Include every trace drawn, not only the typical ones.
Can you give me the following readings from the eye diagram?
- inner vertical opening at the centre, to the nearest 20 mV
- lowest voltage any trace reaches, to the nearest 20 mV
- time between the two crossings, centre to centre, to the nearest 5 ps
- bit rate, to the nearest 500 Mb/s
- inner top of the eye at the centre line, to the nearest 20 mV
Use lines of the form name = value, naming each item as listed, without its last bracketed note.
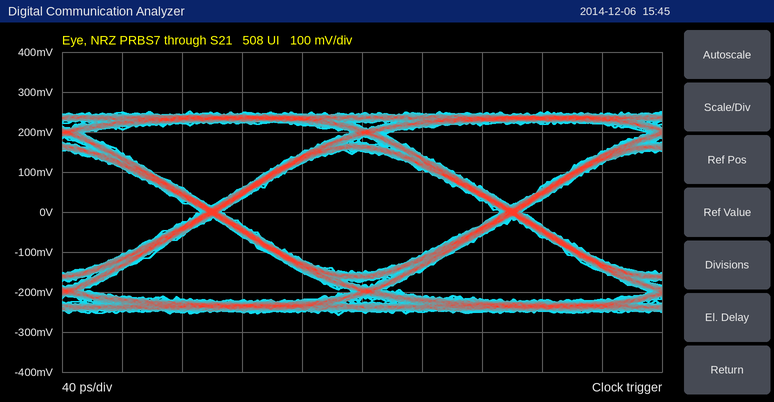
inner vertical opening at the centre, to the nearest 20 mV = 300 mV
lowest voltage any trace reaches, to the nearest 20 mV = -260 mV
time between the two crossings, centre to centre, to the nearest 5 ps = 200 ps
bit rate, to the nearest 500 Mb/s = 5.0 Gb/s
inner top of the eye at the centre line, to the nearest 20 mV = 160 mV
